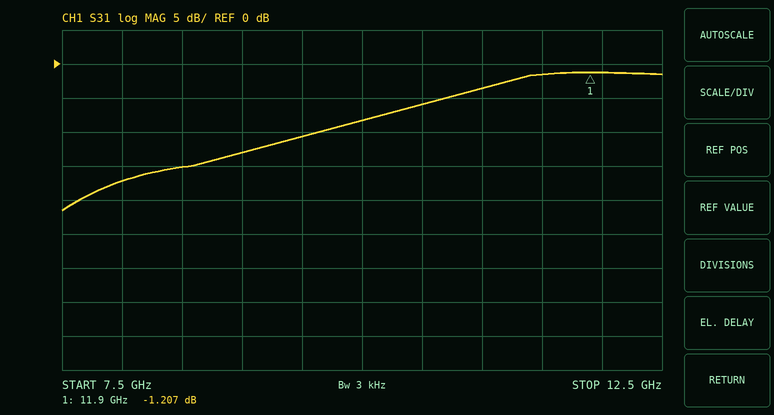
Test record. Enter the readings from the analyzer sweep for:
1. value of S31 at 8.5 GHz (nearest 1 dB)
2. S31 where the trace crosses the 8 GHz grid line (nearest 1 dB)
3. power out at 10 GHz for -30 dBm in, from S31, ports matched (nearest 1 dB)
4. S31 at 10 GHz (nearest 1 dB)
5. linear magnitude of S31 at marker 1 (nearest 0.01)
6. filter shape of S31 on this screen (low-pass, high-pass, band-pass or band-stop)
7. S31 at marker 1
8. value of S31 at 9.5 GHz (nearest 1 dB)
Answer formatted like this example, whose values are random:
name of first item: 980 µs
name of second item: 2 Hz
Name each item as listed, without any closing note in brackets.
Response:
value of S31 at 8.5 GHz: -15 dB
S31 where the trace crosses the 8 GHz grid line: -17 dB
power out at 10 GHz for -30 dBm in, from S31, ports matched: -38 dBm
S31 at 10 GHz: -8 dB
linear magnitude of S31 at marker 1: 0.87
filter shape of S31 on this screen: high-pass
S31 at marker 1: -1.207 dB
value of S31 at 9.5 GHz: -11 dB
